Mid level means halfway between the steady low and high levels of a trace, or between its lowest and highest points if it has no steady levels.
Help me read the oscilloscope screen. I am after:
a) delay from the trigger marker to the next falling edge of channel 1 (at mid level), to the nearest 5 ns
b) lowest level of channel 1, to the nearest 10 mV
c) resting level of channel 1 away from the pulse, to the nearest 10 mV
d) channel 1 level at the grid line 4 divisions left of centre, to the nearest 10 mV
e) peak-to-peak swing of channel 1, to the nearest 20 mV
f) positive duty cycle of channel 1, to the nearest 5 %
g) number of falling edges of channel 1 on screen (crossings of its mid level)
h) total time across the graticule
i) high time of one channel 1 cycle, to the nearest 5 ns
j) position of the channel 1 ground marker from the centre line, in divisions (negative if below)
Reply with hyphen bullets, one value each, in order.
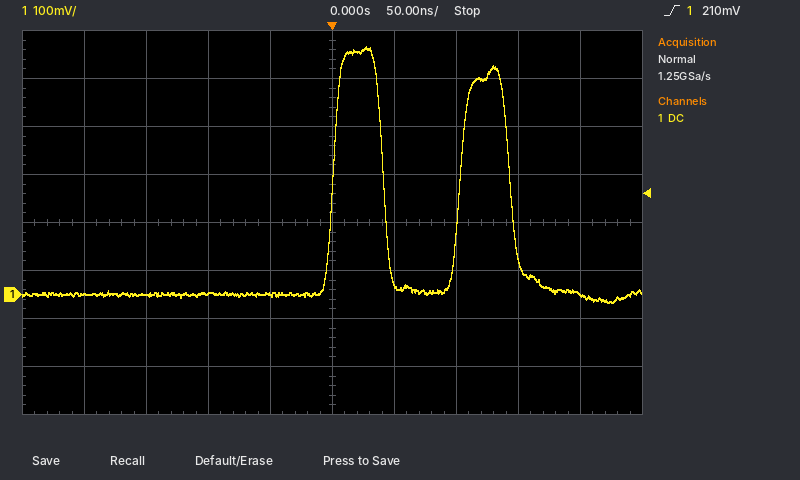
- 40 ns
- -20 mV
- 0 mV
- 0 mV
- 540 mV
- 40 %
- 2
- 500 ns
- 40 ns
- -1.5 div
